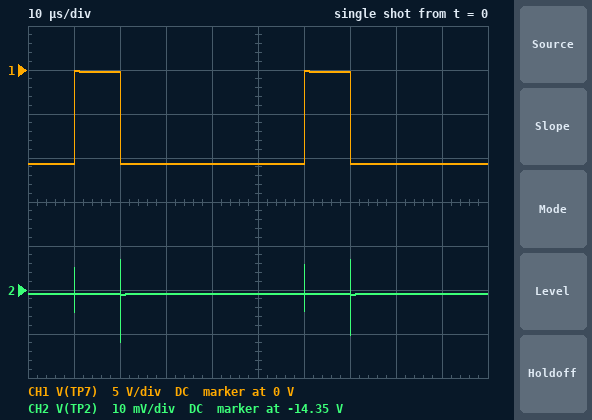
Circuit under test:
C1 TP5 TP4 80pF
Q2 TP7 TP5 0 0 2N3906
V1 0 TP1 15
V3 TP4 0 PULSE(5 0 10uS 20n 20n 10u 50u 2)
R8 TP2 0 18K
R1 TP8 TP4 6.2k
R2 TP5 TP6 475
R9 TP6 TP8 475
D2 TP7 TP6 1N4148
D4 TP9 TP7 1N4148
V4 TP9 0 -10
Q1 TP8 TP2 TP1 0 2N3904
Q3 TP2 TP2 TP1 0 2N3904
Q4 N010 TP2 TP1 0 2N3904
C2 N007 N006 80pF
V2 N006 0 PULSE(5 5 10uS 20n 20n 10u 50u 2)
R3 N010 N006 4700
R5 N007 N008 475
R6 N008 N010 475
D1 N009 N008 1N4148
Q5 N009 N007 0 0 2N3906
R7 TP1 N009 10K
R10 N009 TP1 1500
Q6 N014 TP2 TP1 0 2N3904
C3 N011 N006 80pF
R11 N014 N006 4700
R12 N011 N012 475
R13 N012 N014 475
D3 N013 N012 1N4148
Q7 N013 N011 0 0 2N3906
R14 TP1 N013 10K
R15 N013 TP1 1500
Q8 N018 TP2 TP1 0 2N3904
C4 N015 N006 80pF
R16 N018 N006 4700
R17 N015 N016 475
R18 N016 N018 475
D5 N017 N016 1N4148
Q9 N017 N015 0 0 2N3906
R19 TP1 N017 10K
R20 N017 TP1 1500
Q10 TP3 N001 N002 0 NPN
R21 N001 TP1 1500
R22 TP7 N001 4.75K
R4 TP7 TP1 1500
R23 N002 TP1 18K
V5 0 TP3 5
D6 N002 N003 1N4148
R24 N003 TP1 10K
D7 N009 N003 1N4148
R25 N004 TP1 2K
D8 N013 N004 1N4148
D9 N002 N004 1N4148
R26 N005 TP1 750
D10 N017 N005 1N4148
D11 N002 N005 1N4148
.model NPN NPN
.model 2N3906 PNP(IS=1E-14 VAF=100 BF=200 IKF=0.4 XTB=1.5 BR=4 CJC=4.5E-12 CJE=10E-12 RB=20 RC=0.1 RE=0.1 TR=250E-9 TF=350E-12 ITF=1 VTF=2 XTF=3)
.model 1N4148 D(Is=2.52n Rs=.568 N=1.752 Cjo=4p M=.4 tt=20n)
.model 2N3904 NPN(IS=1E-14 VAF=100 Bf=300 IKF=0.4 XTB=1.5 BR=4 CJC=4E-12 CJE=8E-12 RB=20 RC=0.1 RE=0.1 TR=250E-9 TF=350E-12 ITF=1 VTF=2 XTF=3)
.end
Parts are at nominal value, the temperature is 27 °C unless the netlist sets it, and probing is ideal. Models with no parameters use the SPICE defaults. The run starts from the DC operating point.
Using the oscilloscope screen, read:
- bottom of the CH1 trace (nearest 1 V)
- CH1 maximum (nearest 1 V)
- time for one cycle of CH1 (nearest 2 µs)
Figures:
-11 V
0 V
50 µs
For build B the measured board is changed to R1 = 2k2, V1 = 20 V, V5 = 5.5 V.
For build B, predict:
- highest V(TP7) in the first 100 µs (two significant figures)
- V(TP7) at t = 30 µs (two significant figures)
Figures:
-110 mV
-11 V
